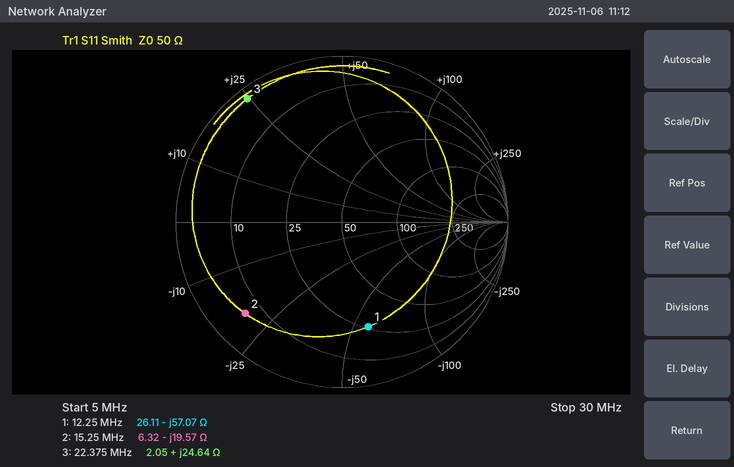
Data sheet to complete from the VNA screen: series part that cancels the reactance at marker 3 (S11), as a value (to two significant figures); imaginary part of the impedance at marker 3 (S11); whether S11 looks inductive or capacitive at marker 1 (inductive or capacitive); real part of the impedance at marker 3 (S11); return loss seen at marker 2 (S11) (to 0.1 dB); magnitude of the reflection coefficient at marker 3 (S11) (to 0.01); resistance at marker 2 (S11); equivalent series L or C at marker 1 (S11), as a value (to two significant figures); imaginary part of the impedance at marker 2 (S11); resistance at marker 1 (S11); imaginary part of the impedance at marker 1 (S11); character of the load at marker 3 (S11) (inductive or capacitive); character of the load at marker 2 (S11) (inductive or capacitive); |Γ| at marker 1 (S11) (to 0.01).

290 pF
+24.64 Ω
capacitive
2.05 Ω
1.9 dB
0.94
6.32 Ω
230 pF
-19.57 Ω
26.11 Ω
-57.07 Ω
inductive
capacitive
0.65
